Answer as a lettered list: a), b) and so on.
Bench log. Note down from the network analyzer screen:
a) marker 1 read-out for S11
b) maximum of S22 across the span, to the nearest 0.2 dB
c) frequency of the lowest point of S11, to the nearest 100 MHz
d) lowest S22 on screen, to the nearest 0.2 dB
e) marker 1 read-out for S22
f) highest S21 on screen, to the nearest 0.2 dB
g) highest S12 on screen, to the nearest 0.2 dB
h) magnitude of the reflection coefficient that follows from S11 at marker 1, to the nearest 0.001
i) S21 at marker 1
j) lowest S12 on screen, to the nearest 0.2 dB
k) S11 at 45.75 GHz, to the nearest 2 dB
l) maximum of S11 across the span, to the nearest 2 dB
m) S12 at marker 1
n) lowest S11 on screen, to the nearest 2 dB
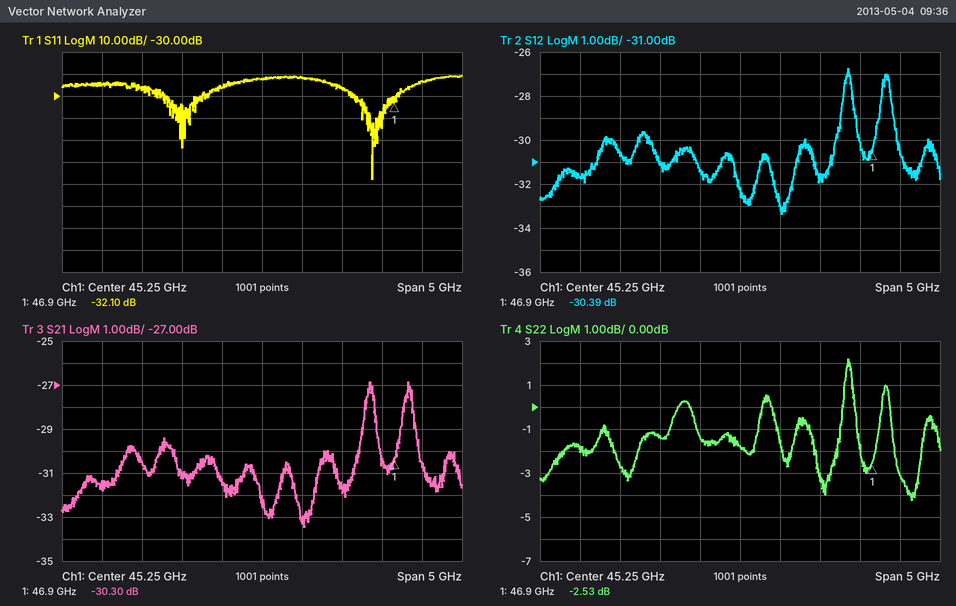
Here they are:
a) -32.10 dB
b) 2.2 dB
c) 46.6 GHz
d) -4.2 dB
e) -2.53 dB
f) -26.8 dB
g) -26.8 dB
h) 0.025
i) -30.30 dB
j) -33.4 dB
k) -22 dB
l) -20 dB
m) -30.39 dB
n) -68 dB
